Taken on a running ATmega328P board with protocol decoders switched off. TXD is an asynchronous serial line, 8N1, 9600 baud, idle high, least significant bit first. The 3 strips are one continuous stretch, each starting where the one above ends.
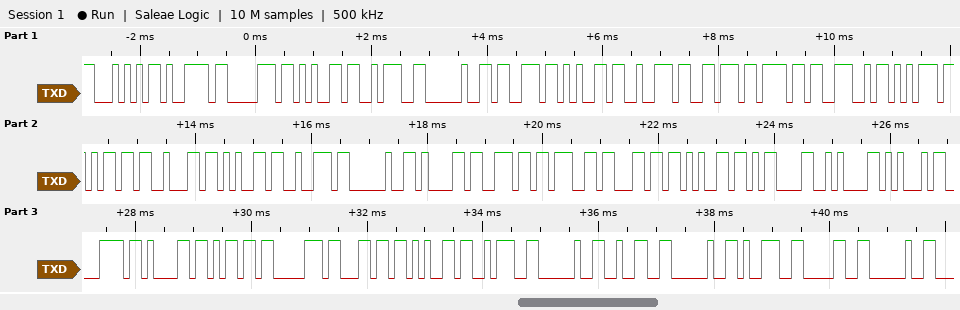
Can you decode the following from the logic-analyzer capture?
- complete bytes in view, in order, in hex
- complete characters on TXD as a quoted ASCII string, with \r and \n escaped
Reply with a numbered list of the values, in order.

1. 54 79 70 65 3A 20 73 65 72 76 6F 4E 75 6D 62 65 72 20 61 6E 67 6C 65 0D 0A 45 78 61 6D 70 6C 65 3A 20 32 20 39 30 20
2. "Type: servoNumber angle\r\nExample: 2 90 "
